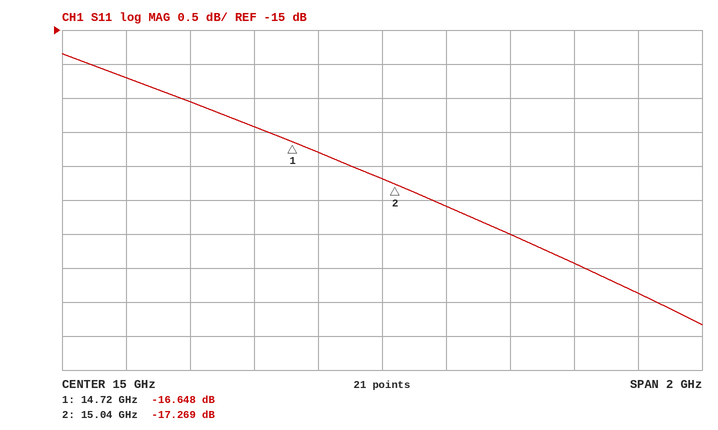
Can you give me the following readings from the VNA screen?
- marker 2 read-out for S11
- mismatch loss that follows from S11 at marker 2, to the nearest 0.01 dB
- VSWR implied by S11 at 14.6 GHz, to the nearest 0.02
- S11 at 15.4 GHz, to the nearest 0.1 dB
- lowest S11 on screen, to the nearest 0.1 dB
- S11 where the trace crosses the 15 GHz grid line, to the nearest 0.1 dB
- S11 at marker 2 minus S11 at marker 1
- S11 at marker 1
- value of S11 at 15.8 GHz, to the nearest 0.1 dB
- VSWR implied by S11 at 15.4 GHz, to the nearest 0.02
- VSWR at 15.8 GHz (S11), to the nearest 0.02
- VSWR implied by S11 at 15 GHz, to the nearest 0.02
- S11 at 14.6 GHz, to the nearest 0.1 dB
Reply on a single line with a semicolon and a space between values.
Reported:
-17.269 dB; 0.08 dB; 1.36; -18.0 dB; -19.3 dB; -17.2 dB; -0.621 dB; -16.648 dB; -18.9 dB; 1.28; 1.26; 1.32; -16.4 dB
